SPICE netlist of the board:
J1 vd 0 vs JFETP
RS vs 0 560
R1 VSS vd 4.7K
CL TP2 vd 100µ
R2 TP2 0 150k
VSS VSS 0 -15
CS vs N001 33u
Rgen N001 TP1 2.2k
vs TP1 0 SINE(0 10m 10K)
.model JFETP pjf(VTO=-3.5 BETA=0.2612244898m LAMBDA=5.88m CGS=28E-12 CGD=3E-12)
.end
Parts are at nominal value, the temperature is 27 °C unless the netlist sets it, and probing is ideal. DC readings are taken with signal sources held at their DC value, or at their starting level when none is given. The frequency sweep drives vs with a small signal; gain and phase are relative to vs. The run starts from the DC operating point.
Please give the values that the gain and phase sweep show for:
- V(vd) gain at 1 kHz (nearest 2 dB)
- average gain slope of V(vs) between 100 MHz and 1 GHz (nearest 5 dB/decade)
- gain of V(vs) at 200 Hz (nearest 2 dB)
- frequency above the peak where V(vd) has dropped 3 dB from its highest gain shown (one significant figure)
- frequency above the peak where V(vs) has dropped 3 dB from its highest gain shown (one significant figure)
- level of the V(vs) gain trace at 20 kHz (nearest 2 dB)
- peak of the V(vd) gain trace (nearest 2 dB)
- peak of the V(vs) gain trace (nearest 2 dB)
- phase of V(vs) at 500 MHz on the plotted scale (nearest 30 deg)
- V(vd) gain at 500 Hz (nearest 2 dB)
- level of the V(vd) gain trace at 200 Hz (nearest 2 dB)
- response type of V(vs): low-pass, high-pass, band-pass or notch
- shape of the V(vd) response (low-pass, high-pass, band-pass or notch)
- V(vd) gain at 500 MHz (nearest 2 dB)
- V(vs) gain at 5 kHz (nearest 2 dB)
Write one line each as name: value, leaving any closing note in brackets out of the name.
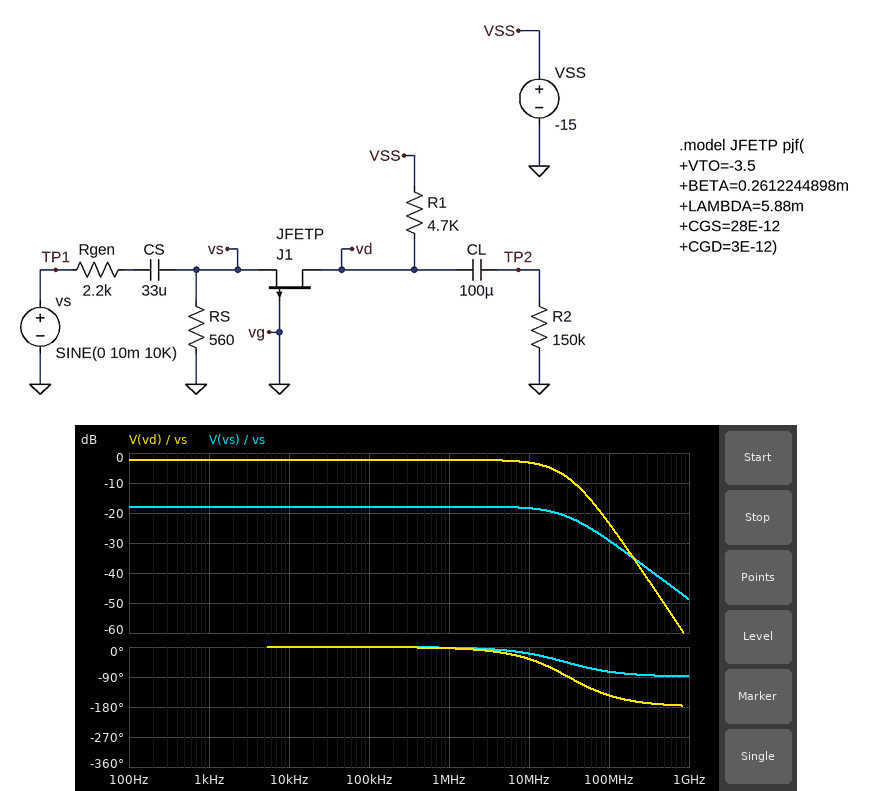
V(vd) gain at 1 kHz: -2 dB
average gain slope of V(vs) between 100 MHz and 1 GHz: -20 dB/decade
gain of V(vs) at 200 Hz: -18 dB
frequency above the peak where V(vd) has dropped 3 dB from its highest gain shown: 20 MHz
frequency above the peak where V(vs) has dropped 3 dB from its highest gain shown: 30 MHz
level of the V(vs) gain trace at 20 kHz: -18 dB
peak of the V(vd) gain trace: -2 dB
peak of the V(vs) gain trace: -18 dB
phase of V(vs) at 500 MHz on the plotted scale: -90 deg
V(vd) gain at 500 Hz: -2 dB
level of the V(vd) gain trace at 200 Hz: -2 dB
response type of V(vs): low-pass, high-pass, band-pass or notch: low-pass
shape of the V(vd) response: low-pass
V(vd) gain at 500 MHz: -50 dB
V(vs) gain at 5 kHz: -18 dB
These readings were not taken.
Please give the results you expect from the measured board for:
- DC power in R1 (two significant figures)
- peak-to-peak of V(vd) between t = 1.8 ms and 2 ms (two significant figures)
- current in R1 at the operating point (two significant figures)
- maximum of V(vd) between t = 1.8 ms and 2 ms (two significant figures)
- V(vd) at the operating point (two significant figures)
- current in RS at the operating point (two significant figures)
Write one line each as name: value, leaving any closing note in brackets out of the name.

DC power in R1: 14 mW
peak-to-peak of V(vd) between t = 1.8 ms and 2 ms: 15 mV
current in R1 at the operating point: 1.7 mA
maximum of V(vd) between t = 1.8 ms and 2 ms: -6.9 V
V(vd) at the operating point: -6.9 V
current in RS at the operating point: 1.7 mA
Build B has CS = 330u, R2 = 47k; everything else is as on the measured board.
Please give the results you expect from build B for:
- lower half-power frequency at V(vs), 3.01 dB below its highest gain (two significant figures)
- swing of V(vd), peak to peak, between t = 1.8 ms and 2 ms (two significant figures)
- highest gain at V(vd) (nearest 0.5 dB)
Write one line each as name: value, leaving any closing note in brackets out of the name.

lower half-power frequency at V(vs), 3.01 dB below its highest gain: 190 mHz
swing of V(vd), peak to peak, between t = 1.8 ms and 2 ms: 14 mV
highest gain at V(vd): -3.0 dB
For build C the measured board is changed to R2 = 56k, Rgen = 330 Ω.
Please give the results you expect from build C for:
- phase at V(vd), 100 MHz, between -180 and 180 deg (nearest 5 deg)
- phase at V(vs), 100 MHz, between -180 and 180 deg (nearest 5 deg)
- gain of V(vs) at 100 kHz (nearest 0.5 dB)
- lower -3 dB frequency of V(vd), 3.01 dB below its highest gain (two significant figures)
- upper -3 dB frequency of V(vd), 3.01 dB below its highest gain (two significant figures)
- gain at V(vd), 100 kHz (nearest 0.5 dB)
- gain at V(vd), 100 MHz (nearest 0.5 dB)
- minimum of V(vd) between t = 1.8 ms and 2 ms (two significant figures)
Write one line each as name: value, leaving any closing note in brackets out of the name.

phase at V(vd), 100 MHz, between -180 and 180 deg: -135 deg
phase at V(vs), 100 MHz, between -180 and 180 deg: -65 deg
gain of V(vs) at 100 kHz: -6.0 dB
lower -3 dB frequency of V(vd), 3.01 dB below its highest gain: 7.4 Hz
upper -3 dB frequency of V(vd), 3.01 dB below its highest gain: 26 MHz
gain at V(vd), 100 kHz: 9.0 dB
gain at V(vd), 100 MHz: -7.5 dB
minimum of V(vd) between t = 1.8 ms and 2 ms: -6.9 V
